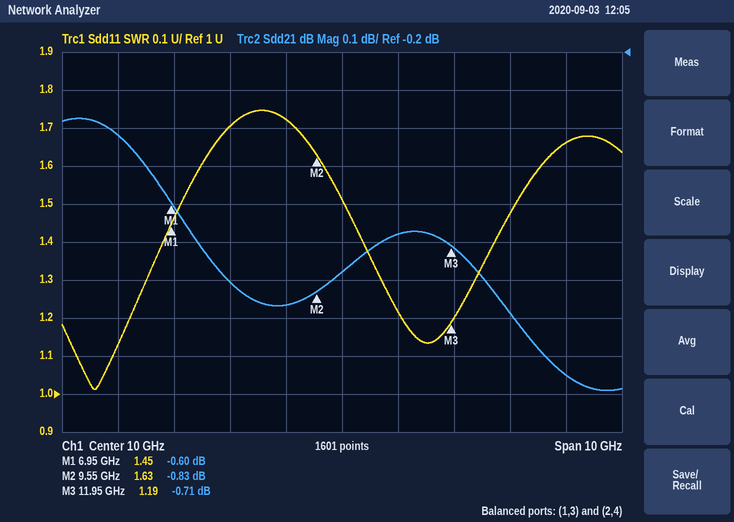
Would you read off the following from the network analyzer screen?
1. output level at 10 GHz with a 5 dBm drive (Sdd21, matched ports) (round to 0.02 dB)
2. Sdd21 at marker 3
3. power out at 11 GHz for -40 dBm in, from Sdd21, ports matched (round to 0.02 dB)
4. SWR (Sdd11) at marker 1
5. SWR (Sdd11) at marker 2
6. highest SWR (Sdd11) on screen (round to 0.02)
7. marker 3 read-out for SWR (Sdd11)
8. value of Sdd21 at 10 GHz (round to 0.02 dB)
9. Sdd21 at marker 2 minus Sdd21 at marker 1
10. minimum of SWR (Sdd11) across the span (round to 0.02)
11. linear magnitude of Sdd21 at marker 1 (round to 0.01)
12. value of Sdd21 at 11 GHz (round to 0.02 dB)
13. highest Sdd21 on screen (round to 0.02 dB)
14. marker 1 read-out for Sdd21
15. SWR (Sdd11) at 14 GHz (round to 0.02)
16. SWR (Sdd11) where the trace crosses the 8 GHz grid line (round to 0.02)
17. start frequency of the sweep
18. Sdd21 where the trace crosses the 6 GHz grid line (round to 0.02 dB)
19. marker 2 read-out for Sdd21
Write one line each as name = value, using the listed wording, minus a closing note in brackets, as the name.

output level at 10 GHz with a 5 dBm drive (Sdd21, matched ports) = 4.22 dBm
Sdd21 at marker 3 = -0.71 dB
power out at 11 GHz for -40 dBm in, from Sdd21, ports matched = -40.68 dBm
SWR (Sdd11) at marker 1 = 1.45
SWR (Sdd11) at marker 2 = 1.63
highest SWR (Sdd11) on screen = 1.74
marker 3 read-out for SWR = 1.19
value of Sdd21 at 10 GHz = -0.78 dB
Sdd21 at marker 2 minus Sdd21 at marker 1 = -0.23 dB
minimum of SWR (Sdd11) across the span = 1.02
linear magnitude of Sdd21 at marker 1 = 0.93
value of Sdd21 at 11 GHz = -0.68 dB
highest Sdd21 on screen = -0.38 dB
marker 1 read-out for Sdd21 = -0.60 dB
SWR (Sdd11) at 14 GHz = 1.66
SWR (Sdd11) where the trace crosses the 8 GHz grid line = 1.70
start frequency of the sweep = 5 GHz
Sdd21 where the trace crosses the 6 GHz grid line = -0.42 dB
marker 2 read-out for Sdd21 = -0.83 dB
